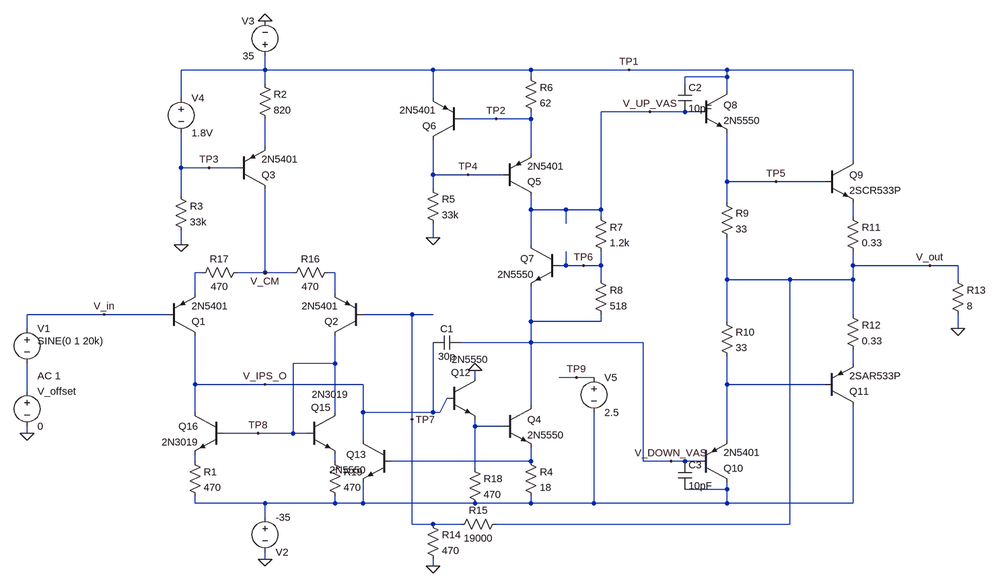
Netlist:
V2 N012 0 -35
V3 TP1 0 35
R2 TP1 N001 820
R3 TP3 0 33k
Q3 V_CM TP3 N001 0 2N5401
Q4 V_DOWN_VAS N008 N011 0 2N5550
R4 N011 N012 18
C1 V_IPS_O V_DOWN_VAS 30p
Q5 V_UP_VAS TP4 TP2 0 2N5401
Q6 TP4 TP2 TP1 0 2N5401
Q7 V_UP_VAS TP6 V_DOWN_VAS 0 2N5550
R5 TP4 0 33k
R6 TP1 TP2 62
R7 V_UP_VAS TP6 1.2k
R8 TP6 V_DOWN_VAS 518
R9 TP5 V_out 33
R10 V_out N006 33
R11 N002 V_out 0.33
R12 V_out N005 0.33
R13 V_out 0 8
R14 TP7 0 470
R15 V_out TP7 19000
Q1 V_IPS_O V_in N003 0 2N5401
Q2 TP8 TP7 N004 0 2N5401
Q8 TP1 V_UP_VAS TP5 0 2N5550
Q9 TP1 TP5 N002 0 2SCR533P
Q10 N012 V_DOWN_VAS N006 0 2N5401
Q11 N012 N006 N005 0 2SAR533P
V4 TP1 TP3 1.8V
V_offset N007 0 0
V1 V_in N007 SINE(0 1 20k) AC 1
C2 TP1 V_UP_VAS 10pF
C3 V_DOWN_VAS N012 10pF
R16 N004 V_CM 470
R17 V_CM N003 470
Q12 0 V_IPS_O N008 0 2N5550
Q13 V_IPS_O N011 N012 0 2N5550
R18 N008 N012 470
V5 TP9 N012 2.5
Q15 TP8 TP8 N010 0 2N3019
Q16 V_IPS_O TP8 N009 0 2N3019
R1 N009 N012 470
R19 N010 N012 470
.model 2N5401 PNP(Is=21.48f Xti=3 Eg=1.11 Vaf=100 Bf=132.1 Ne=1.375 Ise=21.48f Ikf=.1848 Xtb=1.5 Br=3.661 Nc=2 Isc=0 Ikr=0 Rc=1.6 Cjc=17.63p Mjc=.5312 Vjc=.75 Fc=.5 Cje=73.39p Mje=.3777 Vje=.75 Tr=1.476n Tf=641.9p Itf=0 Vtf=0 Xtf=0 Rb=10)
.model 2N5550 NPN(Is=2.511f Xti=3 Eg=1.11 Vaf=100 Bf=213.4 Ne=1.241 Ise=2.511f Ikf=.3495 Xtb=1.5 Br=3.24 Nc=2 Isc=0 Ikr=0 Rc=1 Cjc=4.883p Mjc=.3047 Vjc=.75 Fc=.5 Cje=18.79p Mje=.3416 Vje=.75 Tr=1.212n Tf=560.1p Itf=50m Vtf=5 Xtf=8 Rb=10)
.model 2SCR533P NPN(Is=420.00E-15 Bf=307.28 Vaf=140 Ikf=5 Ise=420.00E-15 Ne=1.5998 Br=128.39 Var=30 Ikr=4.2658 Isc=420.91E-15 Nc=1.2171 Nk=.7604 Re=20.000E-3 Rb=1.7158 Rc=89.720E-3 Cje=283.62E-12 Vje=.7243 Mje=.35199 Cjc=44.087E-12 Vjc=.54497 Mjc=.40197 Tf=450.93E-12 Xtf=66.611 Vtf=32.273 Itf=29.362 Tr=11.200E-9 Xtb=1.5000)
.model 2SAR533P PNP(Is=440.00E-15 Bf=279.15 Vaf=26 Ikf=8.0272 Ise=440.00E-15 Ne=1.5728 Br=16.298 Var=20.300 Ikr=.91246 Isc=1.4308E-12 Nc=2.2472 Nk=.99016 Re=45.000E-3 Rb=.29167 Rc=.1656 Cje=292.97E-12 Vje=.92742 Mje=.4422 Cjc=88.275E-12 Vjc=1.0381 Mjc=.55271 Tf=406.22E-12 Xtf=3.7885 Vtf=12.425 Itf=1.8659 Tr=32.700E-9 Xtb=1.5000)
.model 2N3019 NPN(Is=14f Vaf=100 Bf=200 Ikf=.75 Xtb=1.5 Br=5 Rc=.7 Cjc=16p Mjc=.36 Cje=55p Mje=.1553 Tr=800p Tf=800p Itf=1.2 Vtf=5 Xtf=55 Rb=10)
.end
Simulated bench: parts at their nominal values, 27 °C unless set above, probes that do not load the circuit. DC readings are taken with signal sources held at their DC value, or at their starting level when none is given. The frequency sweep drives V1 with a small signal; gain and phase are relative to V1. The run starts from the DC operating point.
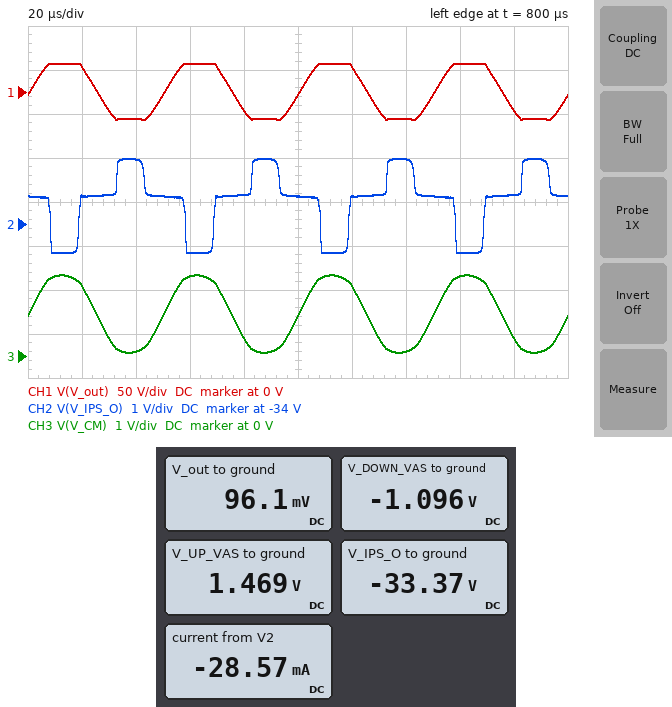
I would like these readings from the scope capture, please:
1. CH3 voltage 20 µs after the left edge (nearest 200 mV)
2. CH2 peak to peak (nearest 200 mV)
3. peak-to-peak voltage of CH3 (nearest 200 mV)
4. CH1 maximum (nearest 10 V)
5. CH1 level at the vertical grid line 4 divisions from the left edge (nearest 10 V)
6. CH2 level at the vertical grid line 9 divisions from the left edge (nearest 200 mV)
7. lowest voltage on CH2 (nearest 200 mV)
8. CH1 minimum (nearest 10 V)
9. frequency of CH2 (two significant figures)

1.6 V
2.2 V
1.8 V
30 V
-20 V
-33.4 V
-34.6 V
-30 V
20 kHz
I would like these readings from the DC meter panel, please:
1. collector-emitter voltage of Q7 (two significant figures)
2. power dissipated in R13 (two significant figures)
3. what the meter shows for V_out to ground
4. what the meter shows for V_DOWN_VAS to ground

2.6 V
1.2 mW
96.1 mV
-1.096 V
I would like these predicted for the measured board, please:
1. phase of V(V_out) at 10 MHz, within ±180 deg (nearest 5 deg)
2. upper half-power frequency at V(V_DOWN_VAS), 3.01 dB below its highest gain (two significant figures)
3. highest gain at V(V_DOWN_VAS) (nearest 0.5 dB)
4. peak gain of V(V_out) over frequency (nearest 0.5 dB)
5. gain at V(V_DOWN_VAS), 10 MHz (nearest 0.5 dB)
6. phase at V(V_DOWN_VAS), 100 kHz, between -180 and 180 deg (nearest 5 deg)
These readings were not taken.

-160 deg
190 kHz
35.0 dB
32.5 dB
-2.5 dB
-30 deg
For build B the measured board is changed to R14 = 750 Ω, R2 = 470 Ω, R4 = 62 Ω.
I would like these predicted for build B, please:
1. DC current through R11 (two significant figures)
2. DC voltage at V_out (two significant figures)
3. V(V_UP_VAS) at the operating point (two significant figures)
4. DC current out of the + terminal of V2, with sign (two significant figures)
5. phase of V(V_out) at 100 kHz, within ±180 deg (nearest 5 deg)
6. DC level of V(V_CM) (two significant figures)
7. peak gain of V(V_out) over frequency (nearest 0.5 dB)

150 mA
1.3 V
2.8 V
-27 mA
-20 deg
1.2 V
27.5 dB
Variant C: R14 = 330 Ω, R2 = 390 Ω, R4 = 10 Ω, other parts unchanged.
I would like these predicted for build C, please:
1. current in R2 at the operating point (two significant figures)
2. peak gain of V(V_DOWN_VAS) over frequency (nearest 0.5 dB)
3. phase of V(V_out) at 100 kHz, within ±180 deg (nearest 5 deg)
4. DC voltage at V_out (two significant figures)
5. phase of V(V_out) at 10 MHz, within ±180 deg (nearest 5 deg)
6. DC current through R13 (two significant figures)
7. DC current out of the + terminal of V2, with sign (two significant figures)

2.9 mA
37.0 dB
-35 deg
-190 mV
-145 deg
24 mA
-53 mA
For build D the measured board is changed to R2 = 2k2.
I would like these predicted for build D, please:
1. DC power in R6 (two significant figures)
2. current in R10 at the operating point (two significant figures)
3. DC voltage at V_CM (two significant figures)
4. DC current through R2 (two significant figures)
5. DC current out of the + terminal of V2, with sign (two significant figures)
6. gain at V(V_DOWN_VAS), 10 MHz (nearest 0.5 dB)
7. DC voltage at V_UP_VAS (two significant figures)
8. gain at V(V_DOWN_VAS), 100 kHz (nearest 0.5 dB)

6.5 mW
14 mA
720 mV
540 µA
-26 mA
-6.5 dB
1.7 V
32.5 dB
